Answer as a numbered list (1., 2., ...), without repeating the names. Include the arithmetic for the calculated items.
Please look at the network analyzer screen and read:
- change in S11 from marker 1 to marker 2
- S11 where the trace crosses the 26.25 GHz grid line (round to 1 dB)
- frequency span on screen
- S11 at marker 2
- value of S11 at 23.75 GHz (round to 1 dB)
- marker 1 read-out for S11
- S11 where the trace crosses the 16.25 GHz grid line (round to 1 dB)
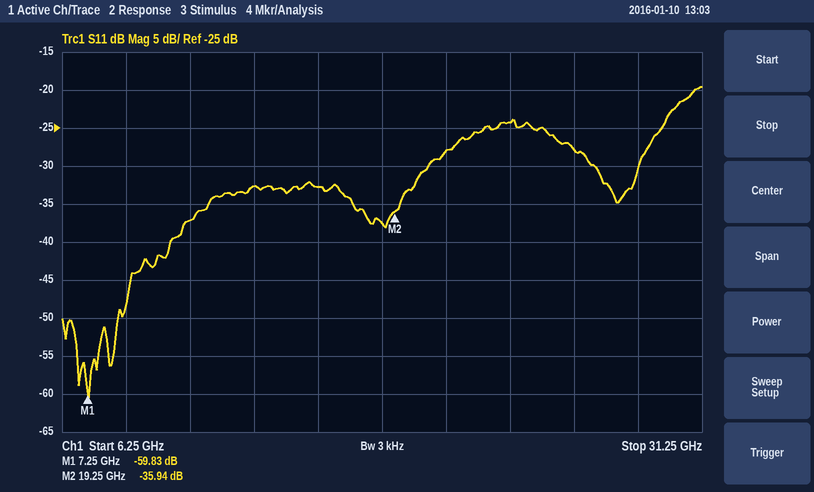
1. -35.94 − (-59.83) = 23.89 dB
2. -28 dB
3. 25 GHz
4. -35.94 dB
5. -24 dB
6. -59.83 dB
7. -33 dB
